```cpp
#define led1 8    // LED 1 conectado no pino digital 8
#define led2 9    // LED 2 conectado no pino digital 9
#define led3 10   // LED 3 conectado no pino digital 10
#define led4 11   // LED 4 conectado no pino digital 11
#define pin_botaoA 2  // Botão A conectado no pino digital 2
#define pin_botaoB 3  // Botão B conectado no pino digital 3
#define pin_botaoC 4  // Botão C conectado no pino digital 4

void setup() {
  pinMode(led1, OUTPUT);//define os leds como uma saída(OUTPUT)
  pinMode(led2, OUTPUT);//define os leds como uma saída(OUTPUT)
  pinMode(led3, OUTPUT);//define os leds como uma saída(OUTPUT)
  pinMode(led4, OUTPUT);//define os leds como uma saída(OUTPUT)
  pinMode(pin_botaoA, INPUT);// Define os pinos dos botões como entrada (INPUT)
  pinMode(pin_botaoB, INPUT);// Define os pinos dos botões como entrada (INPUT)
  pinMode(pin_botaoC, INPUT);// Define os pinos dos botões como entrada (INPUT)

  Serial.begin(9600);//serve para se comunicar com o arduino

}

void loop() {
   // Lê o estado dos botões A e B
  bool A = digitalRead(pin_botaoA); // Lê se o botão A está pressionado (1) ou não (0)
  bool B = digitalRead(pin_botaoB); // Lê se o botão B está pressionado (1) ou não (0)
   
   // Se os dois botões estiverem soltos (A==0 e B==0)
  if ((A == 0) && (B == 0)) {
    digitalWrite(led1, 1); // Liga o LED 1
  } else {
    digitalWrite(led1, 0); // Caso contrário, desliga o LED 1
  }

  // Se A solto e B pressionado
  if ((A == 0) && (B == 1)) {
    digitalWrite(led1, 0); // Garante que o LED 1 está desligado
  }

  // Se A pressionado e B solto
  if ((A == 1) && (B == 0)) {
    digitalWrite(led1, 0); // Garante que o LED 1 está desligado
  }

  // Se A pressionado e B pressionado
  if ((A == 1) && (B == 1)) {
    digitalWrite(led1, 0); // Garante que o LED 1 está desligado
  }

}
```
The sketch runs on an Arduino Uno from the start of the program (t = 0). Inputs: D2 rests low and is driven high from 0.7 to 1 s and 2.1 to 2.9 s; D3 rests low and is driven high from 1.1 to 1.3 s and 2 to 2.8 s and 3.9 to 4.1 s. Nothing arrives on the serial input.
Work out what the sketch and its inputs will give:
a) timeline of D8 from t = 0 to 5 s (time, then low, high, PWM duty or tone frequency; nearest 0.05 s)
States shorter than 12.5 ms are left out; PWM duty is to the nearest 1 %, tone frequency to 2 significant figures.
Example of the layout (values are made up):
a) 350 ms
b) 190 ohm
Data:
a) 0 s high; 0.7 s low; 1 s high; 1.1 s low; 1.3 s high; 2 s low; 2.9 s high; 3.9 s low; 4.1 s high
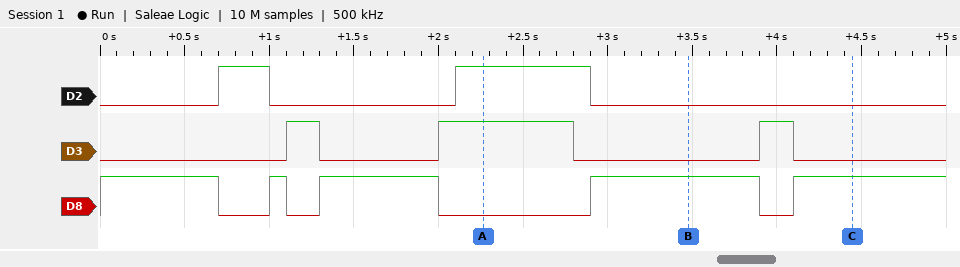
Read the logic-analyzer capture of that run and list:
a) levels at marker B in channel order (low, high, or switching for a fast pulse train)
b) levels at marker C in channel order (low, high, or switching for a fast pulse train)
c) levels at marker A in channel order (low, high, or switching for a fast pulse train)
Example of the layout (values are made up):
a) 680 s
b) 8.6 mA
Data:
a) D2 low, D3 low, D8 high
b) D2 low, D3 low, D8 high
c) D2 high, D3 high, D8 low
